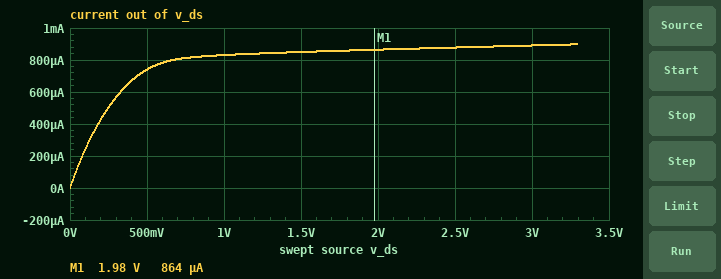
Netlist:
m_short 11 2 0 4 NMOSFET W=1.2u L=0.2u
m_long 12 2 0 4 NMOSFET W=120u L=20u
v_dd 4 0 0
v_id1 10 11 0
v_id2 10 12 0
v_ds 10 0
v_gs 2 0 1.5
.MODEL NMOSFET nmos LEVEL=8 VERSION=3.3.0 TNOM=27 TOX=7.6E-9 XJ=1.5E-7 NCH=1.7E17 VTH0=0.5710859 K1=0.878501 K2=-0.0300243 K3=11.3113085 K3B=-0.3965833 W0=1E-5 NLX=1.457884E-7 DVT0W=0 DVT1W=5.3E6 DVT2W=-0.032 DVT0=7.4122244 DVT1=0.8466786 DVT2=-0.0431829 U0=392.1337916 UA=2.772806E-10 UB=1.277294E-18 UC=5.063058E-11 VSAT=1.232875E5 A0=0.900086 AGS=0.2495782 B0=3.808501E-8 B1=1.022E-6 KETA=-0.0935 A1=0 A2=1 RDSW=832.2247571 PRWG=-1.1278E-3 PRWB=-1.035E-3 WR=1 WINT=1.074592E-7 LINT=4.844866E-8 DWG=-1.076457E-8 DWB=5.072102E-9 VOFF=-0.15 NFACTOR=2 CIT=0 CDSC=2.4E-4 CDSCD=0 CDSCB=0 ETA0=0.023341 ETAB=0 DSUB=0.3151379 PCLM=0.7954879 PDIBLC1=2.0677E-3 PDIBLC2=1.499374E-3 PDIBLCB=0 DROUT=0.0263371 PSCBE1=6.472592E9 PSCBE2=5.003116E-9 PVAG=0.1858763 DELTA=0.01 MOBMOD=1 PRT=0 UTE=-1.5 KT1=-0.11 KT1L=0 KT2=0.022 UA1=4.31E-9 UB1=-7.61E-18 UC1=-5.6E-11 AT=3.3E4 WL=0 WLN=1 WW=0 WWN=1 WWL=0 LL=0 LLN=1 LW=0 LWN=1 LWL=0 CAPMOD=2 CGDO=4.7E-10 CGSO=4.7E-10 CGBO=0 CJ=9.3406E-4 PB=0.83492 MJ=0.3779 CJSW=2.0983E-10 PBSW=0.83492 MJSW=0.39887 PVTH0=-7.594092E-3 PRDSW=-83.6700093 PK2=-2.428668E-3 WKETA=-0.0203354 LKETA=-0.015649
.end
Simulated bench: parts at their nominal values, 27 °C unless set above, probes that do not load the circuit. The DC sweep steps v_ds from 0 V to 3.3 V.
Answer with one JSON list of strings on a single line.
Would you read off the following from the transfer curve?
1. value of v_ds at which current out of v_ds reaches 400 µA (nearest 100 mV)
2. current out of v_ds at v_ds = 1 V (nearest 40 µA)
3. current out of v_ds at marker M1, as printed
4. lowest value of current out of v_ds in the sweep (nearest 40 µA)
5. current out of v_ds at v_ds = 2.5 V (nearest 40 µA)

["200 mV", "840 µA", "864 µA", "0 A", "880 µA"]
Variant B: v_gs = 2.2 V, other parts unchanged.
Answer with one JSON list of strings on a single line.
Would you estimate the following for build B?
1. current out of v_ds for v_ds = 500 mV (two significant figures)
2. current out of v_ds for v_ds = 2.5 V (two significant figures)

["1.3 mA", "1.8 mA"]
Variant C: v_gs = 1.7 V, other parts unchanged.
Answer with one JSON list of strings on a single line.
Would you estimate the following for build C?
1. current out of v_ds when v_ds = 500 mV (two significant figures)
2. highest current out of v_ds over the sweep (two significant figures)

["910 µA", "1.1 mA"]
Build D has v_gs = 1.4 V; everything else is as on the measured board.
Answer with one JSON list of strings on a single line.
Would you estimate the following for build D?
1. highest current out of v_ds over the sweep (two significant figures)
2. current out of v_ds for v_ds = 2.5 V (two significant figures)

["790 µA", "770 µA"]
